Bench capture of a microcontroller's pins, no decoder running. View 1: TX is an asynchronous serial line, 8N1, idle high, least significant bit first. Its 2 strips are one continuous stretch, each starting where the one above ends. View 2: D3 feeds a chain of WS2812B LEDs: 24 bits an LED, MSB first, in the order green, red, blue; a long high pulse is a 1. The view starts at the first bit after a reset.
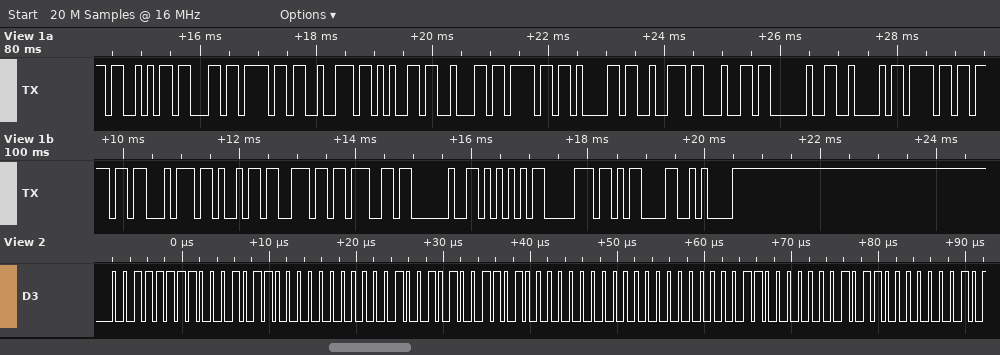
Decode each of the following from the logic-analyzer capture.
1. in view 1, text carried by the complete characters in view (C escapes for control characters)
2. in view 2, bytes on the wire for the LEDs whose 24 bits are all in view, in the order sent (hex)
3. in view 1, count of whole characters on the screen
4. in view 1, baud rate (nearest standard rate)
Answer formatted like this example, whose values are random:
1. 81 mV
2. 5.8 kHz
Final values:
1. "Scoreboard Booting Up\r\n"
2. 3F 16 00 25 34 00 00 30 16
3. 23
4. 9600 baud
